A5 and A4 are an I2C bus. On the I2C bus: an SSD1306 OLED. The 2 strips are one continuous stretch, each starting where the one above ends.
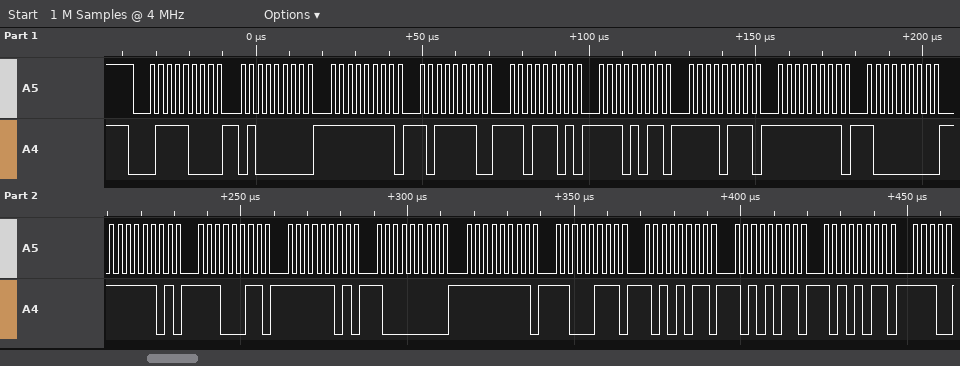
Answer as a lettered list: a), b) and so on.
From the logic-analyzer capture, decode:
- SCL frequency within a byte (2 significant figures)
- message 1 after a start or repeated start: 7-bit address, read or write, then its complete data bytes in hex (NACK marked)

a) 400 kHz
b) 0x3C write: 40 FF BE DD EB F7 FF 80 FD E3 FD 80 FF C7 AB AB AB
